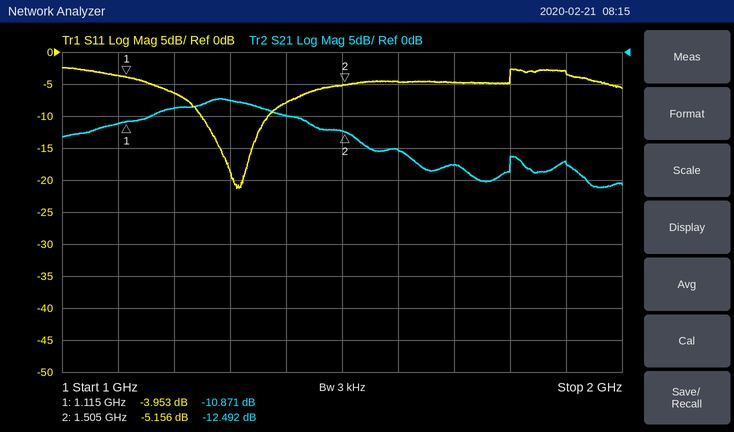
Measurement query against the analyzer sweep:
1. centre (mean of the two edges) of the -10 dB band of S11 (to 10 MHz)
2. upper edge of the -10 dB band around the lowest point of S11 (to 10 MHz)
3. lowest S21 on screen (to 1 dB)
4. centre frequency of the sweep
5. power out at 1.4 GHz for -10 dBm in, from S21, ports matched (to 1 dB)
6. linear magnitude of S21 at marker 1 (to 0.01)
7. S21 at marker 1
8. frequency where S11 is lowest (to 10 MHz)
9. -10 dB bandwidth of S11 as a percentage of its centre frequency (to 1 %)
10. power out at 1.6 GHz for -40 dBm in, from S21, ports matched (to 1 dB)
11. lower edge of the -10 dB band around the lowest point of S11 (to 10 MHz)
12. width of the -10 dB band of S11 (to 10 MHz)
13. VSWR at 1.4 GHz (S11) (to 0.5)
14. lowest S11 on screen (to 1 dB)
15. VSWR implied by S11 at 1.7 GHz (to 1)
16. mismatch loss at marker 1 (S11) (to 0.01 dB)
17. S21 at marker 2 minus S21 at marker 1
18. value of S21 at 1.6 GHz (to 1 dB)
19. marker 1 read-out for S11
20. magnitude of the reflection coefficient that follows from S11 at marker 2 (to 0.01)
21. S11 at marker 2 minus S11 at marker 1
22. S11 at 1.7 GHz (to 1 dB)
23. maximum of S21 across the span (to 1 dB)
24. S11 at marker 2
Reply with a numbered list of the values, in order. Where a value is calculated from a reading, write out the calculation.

1. 1.31 GHz
2. 1.37 GHz
3. -21 dB
4. 1.5 GHz
5. -10 dBm + (-10 dB) = -20 dBm
6. 10^(-10.871/20) ≈ 0.29
7. -10.871 dB
8. 1.31 GHz
9. 120 MHz / 1.31 GHz ≈ 9 %
10. -40 dBm + (-15 dB) = -55 dBm
11. 1.25 GHz
12. 1.37 GHz − 1.25 GHz = 120 MHz
13. |Γ| = 10^(-8/20) = 0.3981; VSWR = (1 + 0.3981)/(1 − 0.3981) ≈ 2.32, so 2.5 to the nearest 0.5
14. -21 dB
15. |Γ| = 10^(-5/20) = 0.5623; VSWR = (1 + 0.5623)/(1 − 0.5623) ≈ 4
16. −10 log10(1 − 10^(-3.953/10)) ≈ 2.24 dB
17. -12.492 − (-10.871) = -1.621 dB
18. -15 dB
19. -3.953 dB
20. 10^(-5.156/20) ≈ 0.55
21. -5.156 − (-3.953) = -1.203 dB
22. -5 dB
23. -7 dB
24. -5.156 dB
